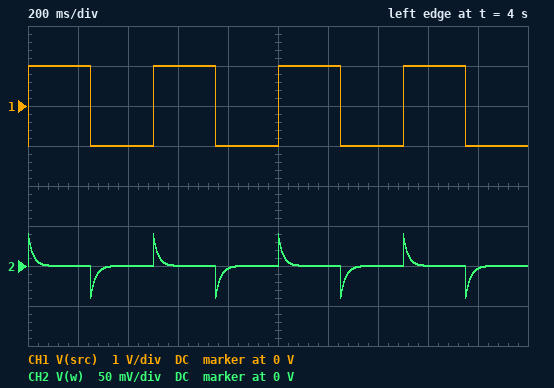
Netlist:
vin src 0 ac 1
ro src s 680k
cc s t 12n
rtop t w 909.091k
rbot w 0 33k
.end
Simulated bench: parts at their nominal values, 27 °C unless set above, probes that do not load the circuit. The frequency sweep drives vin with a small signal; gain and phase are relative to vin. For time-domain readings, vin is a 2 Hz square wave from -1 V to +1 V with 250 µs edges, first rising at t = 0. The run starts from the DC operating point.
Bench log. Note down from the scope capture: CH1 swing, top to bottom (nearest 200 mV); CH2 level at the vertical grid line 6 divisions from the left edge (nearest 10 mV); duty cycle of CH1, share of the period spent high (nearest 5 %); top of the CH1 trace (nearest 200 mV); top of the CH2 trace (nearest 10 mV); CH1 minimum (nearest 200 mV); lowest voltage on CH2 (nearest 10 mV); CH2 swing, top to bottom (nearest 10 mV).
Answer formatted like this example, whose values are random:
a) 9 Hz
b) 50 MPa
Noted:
a) 2.0 V
b) 0 V
c) 50 %
d) 1.0 V
e) 40 mV
f) -1.0 V
g) -40 mV
h) 80 mV
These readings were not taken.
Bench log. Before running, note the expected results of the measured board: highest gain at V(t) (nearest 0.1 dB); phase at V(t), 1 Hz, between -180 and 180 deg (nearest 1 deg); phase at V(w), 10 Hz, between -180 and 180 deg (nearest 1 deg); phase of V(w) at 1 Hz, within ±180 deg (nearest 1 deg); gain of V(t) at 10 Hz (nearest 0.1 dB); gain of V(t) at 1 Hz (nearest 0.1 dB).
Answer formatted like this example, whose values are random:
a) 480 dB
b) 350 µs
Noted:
a) -4.7 dB
b) 83 deg
c) 39 deg
d) 83 deg
e) -6.9 dB
f) -23.0 dB
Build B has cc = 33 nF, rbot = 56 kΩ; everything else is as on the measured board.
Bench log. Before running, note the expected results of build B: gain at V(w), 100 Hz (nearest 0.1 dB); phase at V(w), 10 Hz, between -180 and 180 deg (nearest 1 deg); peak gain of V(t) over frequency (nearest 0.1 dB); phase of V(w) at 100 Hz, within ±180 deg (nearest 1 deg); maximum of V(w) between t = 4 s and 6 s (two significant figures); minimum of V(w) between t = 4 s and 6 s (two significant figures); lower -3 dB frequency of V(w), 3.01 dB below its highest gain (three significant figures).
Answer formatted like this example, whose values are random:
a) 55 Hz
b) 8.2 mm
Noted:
a) -29.4 dB
b) 16 deg
c) -4.6 dB
d) 2 deg
e) 67 mV
f) -67 mV
g) 2.93 Hz
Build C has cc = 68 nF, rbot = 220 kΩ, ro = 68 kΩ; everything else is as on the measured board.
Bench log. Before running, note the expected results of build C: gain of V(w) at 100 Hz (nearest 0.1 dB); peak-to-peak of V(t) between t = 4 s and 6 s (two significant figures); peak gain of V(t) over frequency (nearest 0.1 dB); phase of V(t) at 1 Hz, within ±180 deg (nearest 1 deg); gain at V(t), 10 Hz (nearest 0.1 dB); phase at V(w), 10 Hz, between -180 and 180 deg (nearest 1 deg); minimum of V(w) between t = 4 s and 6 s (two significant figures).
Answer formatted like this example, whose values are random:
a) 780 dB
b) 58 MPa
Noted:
a) -14.7 dB
b) 3.6 V
c) -0.5 dB
d) 63 deg
e) -0.7 dB
f) 11 deg
g) -350 mV
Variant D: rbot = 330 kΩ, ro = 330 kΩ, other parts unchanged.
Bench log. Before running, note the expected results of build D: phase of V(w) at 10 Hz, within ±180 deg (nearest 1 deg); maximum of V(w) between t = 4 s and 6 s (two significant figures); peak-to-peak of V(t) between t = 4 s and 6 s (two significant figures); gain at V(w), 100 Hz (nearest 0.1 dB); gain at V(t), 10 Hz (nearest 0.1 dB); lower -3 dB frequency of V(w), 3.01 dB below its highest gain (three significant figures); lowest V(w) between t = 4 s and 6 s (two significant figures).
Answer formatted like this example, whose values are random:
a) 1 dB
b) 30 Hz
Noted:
a) 40 deg
b) 420 mV
c) 3.1 V
d) -13.6 dB
e) -4.4 dB
f) 8.45 Hz
g) -420 mV
